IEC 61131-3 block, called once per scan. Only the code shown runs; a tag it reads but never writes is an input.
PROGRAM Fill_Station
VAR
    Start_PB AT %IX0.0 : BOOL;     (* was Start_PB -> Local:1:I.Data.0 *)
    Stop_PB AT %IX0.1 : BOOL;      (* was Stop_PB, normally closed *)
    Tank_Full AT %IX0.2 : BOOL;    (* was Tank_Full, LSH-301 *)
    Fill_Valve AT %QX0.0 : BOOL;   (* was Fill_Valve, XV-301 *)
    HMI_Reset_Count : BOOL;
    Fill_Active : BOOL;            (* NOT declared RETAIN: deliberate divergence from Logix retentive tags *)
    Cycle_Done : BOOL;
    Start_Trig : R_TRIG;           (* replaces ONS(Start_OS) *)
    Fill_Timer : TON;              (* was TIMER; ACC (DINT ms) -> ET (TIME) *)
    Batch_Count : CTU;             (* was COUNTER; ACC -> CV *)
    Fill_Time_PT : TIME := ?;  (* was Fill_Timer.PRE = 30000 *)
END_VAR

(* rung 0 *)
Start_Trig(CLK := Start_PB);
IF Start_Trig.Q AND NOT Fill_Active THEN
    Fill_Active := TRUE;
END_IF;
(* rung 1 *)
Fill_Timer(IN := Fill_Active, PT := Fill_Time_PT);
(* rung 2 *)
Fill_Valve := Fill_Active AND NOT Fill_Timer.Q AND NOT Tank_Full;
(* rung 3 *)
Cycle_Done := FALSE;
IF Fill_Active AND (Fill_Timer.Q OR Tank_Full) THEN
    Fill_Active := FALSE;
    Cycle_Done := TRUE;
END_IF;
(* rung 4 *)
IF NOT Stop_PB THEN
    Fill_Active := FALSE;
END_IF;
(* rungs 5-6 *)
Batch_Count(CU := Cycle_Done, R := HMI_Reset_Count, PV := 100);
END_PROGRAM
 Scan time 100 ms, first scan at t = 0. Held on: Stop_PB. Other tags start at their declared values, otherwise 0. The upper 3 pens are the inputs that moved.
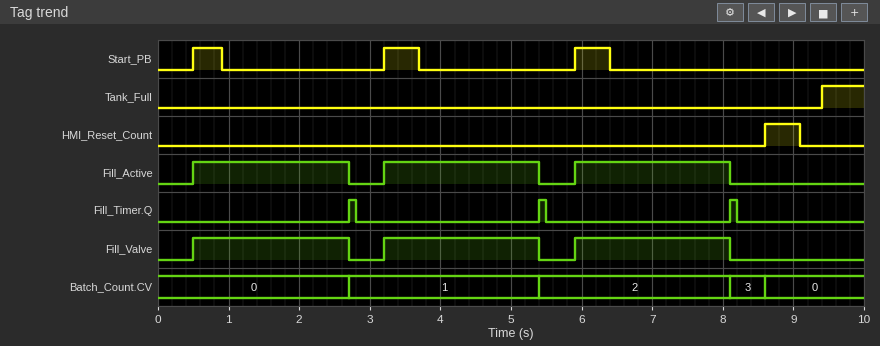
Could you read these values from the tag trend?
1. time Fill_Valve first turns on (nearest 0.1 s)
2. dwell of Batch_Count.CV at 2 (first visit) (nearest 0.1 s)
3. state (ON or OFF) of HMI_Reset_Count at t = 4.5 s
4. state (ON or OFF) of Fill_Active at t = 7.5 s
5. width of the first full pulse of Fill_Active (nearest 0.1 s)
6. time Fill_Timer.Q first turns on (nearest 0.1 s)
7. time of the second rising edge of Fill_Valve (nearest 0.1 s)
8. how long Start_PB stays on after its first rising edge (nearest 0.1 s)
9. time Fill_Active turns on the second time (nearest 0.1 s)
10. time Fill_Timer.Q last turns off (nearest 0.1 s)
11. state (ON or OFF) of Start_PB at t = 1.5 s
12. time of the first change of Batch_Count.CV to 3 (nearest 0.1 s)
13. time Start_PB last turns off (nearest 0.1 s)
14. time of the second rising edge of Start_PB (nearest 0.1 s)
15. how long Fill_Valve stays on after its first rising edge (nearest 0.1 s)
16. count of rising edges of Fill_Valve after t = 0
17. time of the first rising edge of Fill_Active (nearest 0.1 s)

0.5 s
2.7 s
OFF
ON
2.2 s
2.7 s
3.2 s
0.4 s
3.2 s
8.2 s
OFF
8.1 s
6.4 s
3.2 s
2.2 s
3
0.5 s
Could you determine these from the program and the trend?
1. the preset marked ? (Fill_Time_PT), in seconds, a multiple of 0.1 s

2.2 s
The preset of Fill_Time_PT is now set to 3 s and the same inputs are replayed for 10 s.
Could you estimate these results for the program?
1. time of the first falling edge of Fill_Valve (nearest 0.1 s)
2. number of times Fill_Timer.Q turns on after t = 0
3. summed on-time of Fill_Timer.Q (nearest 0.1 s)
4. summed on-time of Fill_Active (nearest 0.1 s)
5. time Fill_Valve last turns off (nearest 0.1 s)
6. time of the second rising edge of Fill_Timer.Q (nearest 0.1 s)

3.5 s
2
0.2 s
6.0 s
8.9 s
8.9 s
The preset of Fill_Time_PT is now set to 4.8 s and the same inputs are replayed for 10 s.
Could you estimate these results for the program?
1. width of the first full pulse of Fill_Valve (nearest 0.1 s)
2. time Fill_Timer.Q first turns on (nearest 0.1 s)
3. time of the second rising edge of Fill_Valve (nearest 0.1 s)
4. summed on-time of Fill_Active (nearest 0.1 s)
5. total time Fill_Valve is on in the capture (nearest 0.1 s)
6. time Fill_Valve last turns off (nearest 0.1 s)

4.8 s
5.3 s
5.9 s
8.3 s
8.3 s
9.4 s
